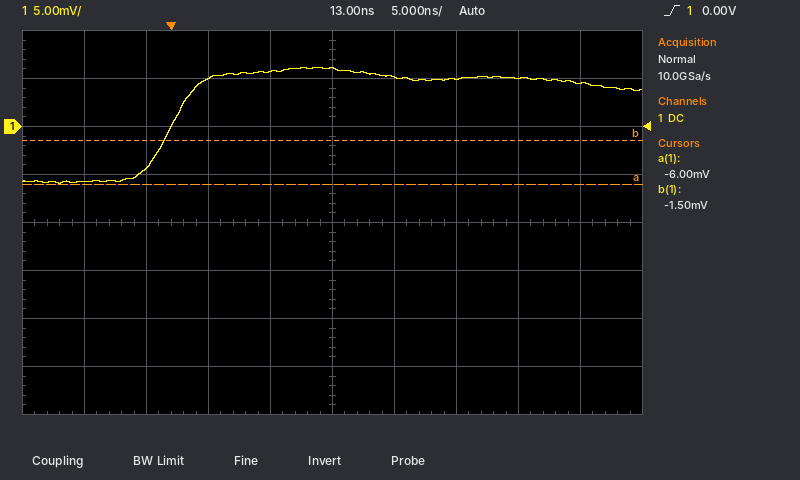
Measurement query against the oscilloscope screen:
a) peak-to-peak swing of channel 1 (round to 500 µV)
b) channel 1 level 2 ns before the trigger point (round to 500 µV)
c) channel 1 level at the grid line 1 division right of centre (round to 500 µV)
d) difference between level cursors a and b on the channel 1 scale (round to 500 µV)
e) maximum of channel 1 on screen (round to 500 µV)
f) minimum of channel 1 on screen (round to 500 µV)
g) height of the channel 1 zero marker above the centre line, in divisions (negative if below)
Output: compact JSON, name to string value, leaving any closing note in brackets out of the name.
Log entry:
{"peak-to-peak swing of channel 1": "12.0 mV", "channel 1 level 2 ns before the trigger point": "-4.5 mV", "channel 1 level at the grid line 1 division right of centre": "5.0 mV", "difference between level cursors a and b on the channel 1 scale": "4.5 mV", "maximum of channel 1 on screen": "6.0 mV", "minimum of channel 1 on screen": "-6.0 mV", "height of the channel 1 zero marker above the centre line, in divisions": "+2.0 div"}
